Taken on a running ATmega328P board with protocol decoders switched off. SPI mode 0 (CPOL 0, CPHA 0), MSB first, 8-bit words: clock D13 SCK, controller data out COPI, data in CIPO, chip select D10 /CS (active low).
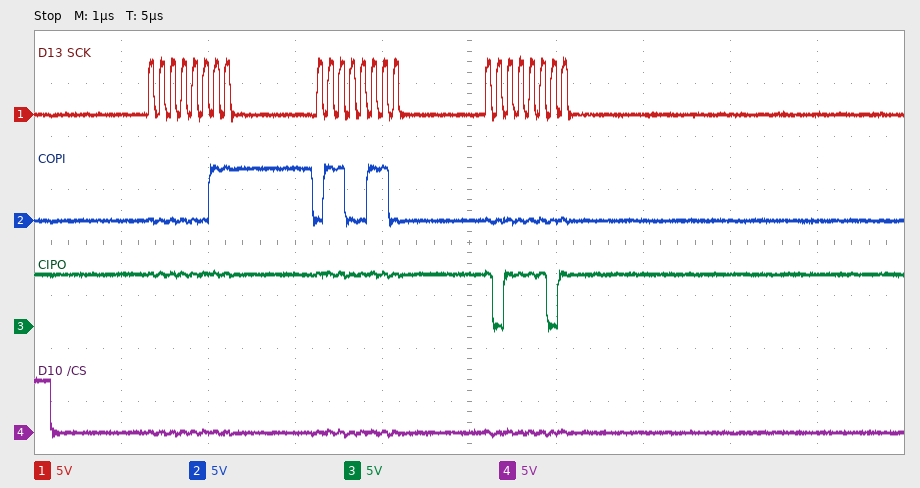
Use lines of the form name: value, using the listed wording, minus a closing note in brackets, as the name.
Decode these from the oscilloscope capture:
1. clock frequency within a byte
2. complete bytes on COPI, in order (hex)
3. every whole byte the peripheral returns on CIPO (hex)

clock frequency within a byte: 8 MHz
complete bytes on COPI, in order: 0x03 0x66 0x00
every whole byte the peripheral returns on CIPO: 0xFF 0xFF 0xBD
